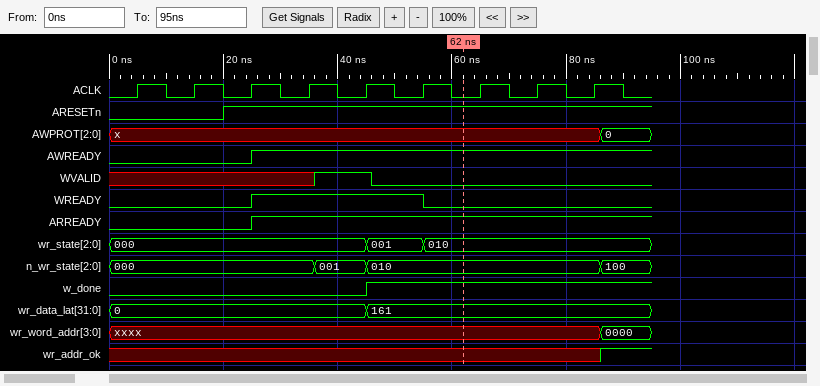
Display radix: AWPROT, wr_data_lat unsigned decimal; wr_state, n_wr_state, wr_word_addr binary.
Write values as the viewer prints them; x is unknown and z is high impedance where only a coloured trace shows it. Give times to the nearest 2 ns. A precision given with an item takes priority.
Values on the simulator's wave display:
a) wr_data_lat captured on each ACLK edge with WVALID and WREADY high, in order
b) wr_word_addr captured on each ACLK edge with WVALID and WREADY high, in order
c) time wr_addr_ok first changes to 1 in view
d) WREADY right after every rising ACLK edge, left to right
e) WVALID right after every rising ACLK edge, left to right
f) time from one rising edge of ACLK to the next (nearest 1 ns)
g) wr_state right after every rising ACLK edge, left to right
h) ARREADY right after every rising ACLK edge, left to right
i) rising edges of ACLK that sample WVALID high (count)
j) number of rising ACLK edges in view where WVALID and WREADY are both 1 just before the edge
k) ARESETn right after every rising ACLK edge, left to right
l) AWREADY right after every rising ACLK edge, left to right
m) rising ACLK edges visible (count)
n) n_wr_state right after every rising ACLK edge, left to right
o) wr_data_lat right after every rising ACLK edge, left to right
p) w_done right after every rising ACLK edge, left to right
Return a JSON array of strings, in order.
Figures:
["0", "xxxx", "86 ns", "0 0 1 1 1 0 0 0 0", "x x x x 1 0 0 0 0", "10 ns", "000, 000, 000, 000, 001, 010, 010, 010, 010", "0 0 1 1 1 1 1 1 1", "1", "1", "0 0 1 1 1 1 1 1 1", "0 0 1 1 1 1 1 1 1", "9", "000, 000, 000, 000, 010, 010, 010, 010, 010", "0, 0, 0, 0, 161, 161, 161, 161, 161", "0 0 0 0 1 1 1 1 1"]
